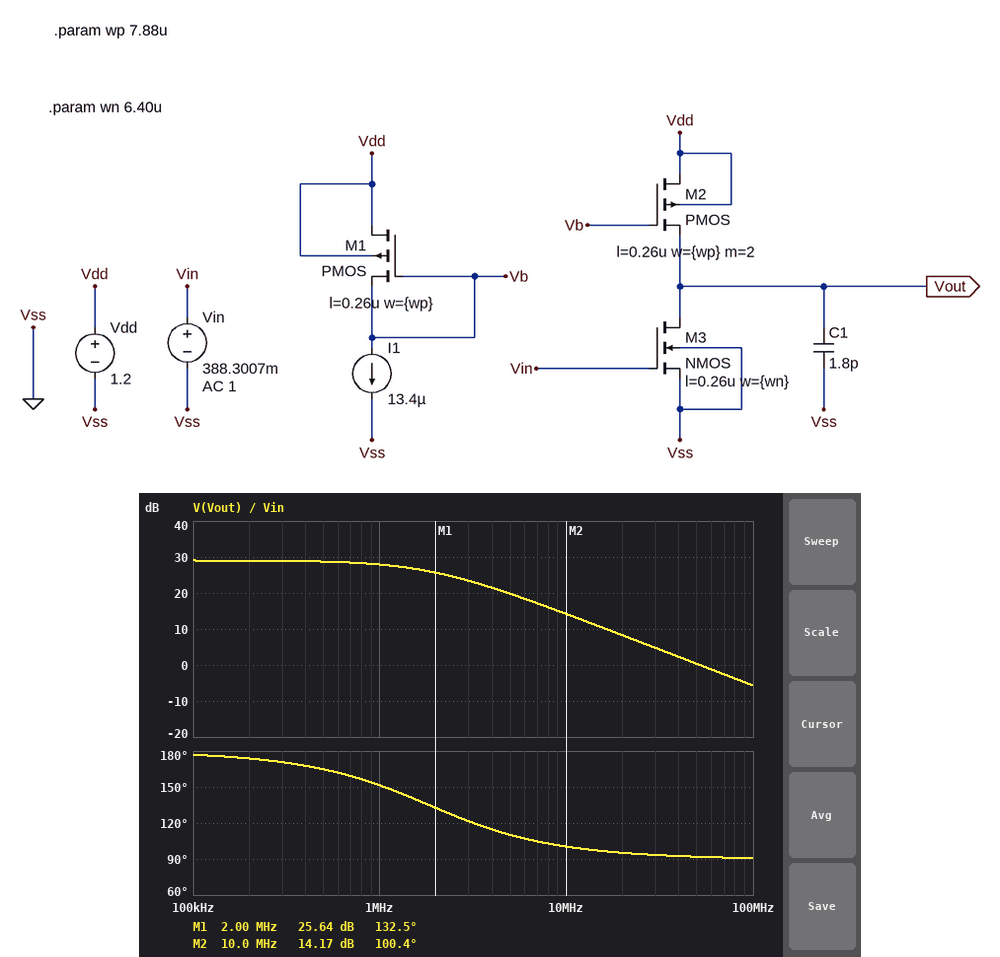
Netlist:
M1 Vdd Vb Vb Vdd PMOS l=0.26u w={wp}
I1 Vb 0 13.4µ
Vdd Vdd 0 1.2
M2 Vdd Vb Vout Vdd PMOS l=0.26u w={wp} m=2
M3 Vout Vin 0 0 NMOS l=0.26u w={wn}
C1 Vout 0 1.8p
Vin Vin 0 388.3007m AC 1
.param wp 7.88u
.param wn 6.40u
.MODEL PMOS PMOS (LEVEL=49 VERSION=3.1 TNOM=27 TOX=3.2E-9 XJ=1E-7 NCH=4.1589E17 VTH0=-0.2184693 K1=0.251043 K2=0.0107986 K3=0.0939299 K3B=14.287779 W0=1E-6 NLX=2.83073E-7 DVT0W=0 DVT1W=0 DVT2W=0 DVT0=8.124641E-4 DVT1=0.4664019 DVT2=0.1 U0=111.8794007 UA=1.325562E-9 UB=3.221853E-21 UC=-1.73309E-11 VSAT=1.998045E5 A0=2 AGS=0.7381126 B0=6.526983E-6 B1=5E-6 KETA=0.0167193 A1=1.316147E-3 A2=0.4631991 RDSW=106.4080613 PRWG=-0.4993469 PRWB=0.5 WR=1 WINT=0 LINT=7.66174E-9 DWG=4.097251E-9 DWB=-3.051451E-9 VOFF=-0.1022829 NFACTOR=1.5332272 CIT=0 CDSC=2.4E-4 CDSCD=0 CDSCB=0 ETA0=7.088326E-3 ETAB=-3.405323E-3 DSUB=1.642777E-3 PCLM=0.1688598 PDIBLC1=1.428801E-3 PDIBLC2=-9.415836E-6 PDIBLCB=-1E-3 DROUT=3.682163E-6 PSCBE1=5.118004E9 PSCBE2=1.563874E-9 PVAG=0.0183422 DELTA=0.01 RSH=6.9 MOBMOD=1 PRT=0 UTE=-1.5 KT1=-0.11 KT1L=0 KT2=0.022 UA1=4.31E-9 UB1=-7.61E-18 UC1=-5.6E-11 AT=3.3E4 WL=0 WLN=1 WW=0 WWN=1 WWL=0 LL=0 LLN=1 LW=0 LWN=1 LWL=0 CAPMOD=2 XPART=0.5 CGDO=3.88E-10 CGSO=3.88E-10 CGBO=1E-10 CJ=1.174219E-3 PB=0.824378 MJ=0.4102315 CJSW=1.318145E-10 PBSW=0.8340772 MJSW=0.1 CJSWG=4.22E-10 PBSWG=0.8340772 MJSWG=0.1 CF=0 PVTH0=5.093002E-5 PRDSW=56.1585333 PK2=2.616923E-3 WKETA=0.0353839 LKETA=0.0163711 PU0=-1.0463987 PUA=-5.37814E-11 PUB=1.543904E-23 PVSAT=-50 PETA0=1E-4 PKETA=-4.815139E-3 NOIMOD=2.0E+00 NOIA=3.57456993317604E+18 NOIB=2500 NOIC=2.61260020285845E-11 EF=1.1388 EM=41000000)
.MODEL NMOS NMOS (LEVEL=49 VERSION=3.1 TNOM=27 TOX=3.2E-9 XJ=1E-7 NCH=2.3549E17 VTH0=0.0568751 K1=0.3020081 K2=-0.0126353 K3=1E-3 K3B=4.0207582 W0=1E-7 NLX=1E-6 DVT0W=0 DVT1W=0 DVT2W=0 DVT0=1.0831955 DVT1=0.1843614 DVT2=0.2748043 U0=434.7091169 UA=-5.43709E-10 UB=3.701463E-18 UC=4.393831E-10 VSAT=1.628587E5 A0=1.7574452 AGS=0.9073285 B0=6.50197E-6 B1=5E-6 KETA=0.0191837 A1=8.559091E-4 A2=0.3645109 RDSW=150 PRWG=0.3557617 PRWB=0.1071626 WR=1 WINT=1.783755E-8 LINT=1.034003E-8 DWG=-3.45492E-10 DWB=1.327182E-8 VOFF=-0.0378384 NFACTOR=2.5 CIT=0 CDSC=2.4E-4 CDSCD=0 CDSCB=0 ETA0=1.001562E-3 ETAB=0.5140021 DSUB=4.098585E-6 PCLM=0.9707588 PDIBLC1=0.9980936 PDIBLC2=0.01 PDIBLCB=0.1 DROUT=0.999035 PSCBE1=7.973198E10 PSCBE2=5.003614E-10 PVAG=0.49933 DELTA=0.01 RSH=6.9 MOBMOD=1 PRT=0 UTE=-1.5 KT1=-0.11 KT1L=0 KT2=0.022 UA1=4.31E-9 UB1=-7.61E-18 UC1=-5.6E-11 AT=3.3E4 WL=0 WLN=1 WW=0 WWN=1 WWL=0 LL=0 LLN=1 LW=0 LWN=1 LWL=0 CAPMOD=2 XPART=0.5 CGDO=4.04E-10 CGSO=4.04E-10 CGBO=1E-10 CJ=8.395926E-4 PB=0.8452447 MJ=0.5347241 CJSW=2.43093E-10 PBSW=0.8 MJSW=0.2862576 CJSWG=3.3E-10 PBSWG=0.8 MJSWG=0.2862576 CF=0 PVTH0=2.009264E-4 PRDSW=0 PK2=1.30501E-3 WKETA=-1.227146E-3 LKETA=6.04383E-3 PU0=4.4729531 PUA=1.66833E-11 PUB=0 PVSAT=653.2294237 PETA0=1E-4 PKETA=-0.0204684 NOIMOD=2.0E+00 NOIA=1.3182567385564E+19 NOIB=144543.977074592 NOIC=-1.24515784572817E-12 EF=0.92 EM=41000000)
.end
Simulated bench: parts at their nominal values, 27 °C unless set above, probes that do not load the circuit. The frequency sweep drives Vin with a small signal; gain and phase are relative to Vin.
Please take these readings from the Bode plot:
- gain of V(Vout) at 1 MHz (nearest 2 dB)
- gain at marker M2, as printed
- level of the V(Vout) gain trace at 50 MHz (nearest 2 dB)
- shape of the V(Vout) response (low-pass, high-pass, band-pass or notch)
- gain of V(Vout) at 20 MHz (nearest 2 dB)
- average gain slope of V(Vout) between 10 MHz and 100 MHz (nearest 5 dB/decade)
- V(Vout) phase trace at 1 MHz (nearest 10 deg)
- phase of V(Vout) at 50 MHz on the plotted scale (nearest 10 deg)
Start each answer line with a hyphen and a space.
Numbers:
- 28 dB
- 14.17 dB
- 0 dB
- low-pass
- 8 dB
- -20 dB/decade
- 150 deg
- 90 deg
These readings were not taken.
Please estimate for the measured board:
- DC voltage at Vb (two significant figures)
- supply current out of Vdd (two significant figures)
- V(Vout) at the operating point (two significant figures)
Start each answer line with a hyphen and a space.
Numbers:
- 800 mV
- 42 µA
- 610 mV
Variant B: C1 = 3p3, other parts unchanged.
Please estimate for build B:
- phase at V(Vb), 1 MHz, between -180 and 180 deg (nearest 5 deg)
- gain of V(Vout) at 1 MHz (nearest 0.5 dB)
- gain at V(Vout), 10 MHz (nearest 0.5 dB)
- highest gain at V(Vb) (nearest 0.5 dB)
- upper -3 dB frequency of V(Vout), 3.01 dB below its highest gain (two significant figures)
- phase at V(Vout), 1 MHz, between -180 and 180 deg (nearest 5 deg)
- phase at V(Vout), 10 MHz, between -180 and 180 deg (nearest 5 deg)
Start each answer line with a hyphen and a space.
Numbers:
- -135 deg
- 26.0 dB
- 9.0 dB
- -47.0 dB
- 1.0 MHz
- 135 deg
- 95 deg
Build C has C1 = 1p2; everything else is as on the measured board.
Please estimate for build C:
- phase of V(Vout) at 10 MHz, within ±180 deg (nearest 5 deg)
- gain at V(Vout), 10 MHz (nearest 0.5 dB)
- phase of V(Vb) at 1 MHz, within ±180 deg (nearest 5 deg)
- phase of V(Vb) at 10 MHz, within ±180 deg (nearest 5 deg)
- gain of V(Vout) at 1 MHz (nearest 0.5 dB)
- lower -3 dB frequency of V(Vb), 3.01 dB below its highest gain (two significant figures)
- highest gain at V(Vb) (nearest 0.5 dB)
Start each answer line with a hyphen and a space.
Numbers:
- 105 deg
- 17.5 dB
- -110 deg
- -165 deg
- 28.5 dB
- 2.7 MHz
- -38.5 dB
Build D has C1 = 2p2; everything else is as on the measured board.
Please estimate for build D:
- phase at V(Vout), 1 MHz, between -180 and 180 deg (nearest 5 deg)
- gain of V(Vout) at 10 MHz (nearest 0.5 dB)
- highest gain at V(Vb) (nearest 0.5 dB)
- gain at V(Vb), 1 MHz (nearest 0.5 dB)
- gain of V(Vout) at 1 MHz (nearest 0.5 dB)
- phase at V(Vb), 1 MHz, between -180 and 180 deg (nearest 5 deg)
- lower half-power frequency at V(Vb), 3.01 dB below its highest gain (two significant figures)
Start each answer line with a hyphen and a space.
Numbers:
- 145 deg
- 12.5 dB
- -43.5 dB
- -49.0 dB
- 27.5 dB
- -125 deg
- 1.5 MHz
